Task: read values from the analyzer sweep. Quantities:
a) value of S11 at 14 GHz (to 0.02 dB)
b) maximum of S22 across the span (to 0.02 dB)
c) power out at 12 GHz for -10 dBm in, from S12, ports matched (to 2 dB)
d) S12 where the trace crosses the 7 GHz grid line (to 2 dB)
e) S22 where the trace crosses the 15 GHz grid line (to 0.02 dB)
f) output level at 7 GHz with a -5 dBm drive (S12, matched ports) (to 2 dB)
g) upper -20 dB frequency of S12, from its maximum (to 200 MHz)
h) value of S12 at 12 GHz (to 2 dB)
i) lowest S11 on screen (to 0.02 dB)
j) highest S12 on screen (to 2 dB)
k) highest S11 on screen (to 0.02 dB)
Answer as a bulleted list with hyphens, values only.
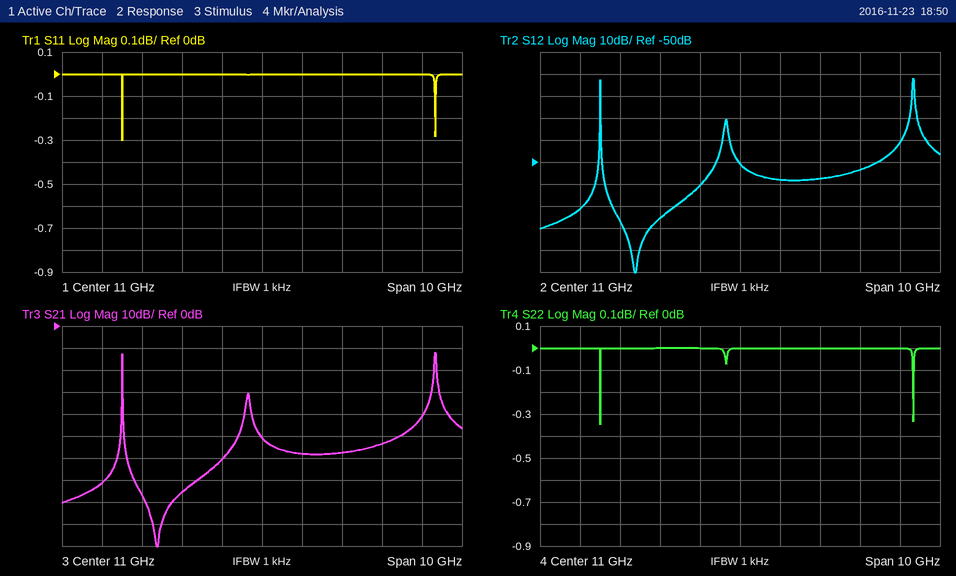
- 0.00 dB
- 0.00 dB
- -68 dBm
- -72 dB
- 0.00 dB
- -76 dBm
- 15.4 GHz
- -58 dB
- -0.30 dB
- -12 dB
- 0.00 dB
